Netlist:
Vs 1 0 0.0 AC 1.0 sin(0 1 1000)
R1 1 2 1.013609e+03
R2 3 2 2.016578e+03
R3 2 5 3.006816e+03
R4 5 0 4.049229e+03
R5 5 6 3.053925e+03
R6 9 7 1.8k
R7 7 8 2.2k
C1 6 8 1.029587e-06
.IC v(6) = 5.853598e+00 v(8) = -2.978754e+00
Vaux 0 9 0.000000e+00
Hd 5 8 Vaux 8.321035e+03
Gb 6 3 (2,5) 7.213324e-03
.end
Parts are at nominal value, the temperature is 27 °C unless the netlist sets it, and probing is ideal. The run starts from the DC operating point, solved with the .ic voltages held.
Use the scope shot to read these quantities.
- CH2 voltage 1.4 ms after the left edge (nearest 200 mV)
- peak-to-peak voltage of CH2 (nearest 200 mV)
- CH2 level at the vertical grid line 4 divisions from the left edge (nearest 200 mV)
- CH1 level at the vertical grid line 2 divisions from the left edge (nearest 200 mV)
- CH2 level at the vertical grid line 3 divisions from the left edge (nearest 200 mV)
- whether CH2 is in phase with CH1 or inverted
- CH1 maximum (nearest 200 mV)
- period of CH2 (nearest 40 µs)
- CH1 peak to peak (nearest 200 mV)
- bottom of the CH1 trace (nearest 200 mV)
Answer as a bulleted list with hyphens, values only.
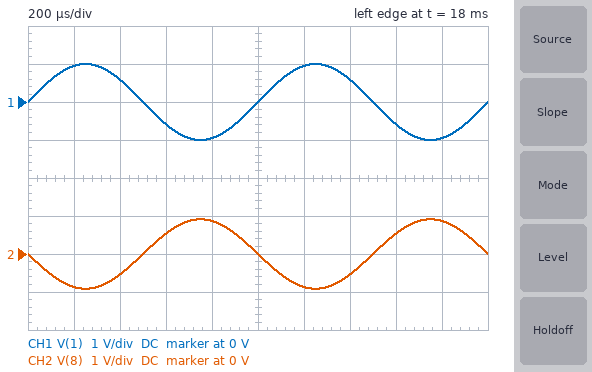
- -600 mV
- 1.8 V
- 800 mV
- 600 mV
- 600 mV
- inverted
- 1.0 V
- 1.00 ms
- 2.0 V
- -1.0 V
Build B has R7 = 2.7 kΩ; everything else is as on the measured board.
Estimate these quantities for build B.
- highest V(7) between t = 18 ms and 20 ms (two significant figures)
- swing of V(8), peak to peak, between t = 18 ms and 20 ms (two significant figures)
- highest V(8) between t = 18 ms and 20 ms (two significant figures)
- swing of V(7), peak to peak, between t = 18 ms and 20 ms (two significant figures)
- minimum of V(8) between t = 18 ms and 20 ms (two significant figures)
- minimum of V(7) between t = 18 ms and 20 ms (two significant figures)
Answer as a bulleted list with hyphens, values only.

- 480 mV
- 2.4 V
- 1.2 V
- 950 mV
- -1.2 V
- -480 mV
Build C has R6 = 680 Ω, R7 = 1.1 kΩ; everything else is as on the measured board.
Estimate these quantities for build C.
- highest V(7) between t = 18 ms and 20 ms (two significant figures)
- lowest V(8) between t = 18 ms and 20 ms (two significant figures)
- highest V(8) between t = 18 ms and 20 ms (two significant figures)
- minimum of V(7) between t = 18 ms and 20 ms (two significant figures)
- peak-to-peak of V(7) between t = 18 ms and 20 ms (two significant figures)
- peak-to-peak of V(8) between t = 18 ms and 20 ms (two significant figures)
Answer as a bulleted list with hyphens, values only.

- 96 mV
- -250 mV
- 250 mV
- -96 mV
- 190 mV
- 500 mV
